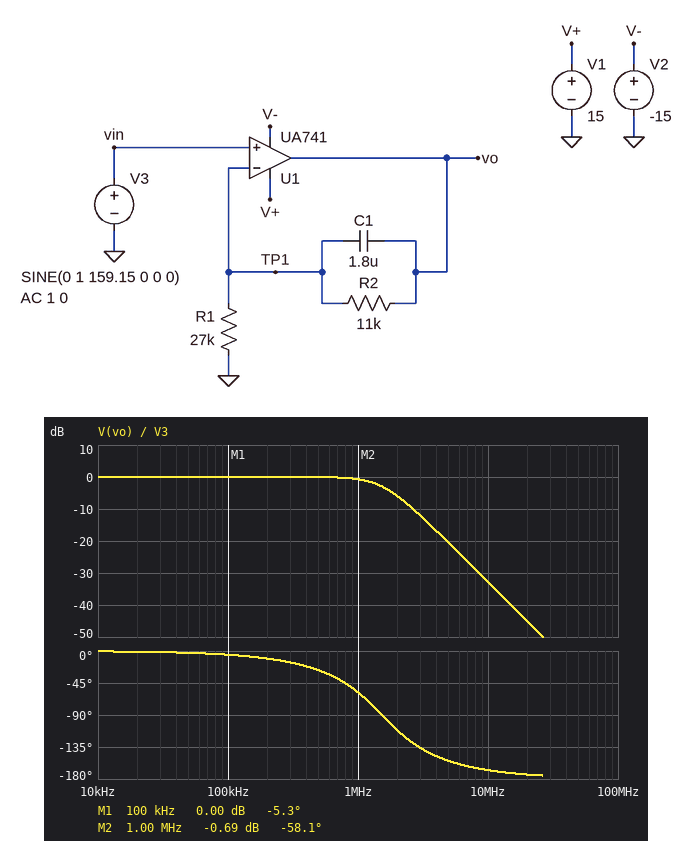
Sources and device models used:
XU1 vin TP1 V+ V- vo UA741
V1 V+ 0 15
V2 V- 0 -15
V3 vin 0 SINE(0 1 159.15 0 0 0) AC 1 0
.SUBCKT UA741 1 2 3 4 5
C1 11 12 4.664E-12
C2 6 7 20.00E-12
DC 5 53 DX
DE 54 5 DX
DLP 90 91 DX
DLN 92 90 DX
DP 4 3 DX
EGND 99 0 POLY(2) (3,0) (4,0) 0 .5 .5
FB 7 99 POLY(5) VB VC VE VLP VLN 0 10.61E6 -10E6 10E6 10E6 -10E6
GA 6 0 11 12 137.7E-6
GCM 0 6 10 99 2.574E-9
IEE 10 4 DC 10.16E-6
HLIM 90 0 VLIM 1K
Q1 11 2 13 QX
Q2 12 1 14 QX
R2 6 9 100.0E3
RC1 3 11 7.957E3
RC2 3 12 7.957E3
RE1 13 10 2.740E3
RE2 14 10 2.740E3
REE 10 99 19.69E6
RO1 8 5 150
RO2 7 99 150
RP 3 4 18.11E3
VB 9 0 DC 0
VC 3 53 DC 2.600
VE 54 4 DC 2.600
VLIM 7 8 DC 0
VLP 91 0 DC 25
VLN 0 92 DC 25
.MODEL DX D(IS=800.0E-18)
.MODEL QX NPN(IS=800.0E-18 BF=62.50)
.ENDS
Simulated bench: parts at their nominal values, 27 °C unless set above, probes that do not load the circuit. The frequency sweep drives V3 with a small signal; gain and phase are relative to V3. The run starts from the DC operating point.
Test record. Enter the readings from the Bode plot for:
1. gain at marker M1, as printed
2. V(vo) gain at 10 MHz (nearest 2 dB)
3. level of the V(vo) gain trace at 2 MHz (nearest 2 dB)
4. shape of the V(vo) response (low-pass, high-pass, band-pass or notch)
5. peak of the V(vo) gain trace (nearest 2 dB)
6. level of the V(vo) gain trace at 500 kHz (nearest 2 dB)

0.00 dB
-32 dB
-6 dB
low-pass
0 dB
0 dB
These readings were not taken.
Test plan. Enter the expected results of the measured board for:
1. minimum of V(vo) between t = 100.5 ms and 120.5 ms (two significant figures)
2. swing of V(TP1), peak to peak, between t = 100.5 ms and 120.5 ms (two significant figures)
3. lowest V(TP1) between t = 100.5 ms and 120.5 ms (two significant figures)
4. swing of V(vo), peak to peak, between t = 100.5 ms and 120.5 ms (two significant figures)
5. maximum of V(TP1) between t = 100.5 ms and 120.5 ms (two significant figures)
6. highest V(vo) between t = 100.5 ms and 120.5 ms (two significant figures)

-1.0 V
2.0 V
-1.0 V
2.0 V
1.0 V
1.0 V
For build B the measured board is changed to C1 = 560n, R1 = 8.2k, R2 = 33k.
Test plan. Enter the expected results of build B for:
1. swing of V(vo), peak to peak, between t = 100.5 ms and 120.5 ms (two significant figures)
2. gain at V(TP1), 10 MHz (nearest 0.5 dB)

2.1 V
-33.0 dB
